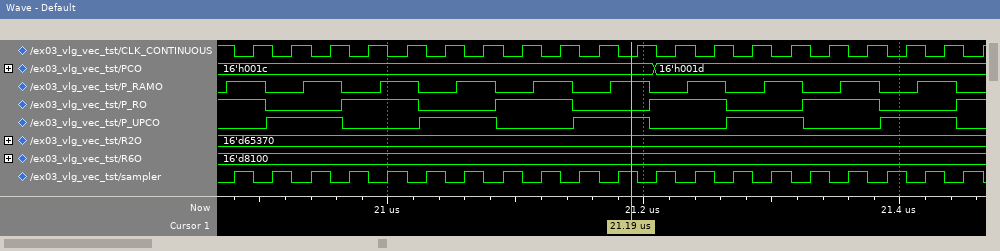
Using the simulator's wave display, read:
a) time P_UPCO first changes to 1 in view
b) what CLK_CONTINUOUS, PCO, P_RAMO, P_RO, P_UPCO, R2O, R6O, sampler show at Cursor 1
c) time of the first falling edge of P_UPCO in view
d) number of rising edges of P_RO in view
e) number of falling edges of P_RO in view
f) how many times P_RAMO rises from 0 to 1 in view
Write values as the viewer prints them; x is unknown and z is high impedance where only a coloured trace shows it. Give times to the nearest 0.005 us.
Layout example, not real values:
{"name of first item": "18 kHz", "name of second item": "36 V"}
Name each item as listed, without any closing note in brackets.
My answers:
{"time P_UPCO first changes to 1 in view": "20.905 us", "what CLK_CONTINUOUS, PCO, P_RAMO, P_RO, P_UPCO, R2O, R6O, sampler show at Cursor 1": "CLK_CONTINUOUS=0, PCO=16'h001c, P_RAMO=1, P_RO=0, P_UPCO=1, R2O=16'd65370, R6O=16'd8100, sampler=1", "time of the first falling edge of P_UPCO in view": "20.965 us", "number of rising edges of P_RO in view": "5", "number of falling edges of P_RO in view": "5", "how many times P_RAMO rises from 0 to 1 in view": "10"}
